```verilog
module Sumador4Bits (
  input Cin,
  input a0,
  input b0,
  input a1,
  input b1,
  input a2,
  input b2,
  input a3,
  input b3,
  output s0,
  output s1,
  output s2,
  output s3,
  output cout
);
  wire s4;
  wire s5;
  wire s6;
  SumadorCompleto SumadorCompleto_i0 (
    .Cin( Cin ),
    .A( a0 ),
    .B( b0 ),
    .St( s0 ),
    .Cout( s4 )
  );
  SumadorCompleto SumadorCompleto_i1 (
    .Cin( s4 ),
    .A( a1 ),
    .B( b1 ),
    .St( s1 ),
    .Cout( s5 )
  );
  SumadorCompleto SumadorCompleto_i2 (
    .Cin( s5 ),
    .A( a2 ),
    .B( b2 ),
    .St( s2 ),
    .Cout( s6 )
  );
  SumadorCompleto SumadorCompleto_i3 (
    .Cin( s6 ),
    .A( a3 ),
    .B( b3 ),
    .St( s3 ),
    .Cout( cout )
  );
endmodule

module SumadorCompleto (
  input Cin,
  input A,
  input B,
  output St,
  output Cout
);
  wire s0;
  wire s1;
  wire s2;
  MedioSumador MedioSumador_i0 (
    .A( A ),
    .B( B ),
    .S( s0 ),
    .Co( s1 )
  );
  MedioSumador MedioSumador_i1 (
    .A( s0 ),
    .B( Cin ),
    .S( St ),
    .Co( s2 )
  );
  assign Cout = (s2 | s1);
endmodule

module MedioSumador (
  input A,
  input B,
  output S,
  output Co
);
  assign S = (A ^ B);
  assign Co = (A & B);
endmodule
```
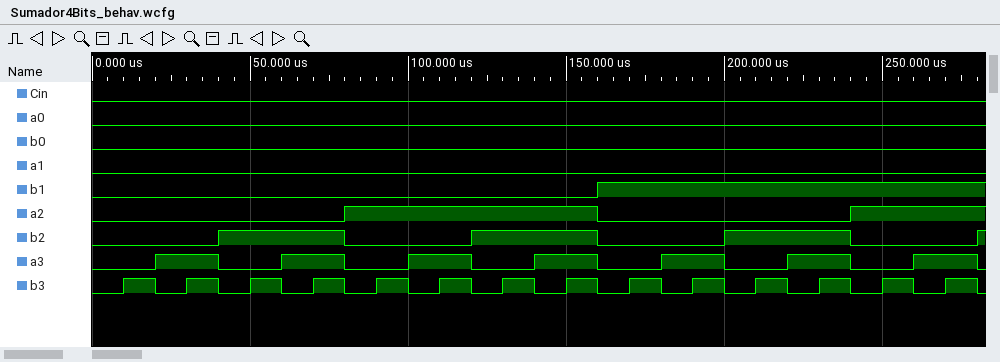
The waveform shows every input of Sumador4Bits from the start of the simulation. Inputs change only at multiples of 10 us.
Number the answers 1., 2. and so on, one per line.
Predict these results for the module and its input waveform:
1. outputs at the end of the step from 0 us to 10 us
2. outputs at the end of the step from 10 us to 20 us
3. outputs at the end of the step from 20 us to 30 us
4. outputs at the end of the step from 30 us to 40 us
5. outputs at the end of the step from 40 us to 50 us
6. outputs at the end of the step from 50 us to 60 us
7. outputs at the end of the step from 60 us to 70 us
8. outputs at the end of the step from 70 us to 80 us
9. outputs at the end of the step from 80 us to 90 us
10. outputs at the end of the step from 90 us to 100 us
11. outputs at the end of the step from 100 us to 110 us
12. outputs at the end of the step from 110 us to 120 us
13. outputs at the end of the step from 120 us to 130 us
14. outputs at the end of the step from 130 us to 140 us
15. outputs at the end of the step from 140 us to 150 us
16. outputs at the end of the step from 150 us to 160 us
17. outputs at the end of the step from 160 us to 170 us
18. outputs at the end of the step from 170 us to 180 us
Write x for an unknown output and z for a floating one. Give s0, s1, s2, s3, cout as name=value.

1. s0=0, s1=0, s2=0, s3=0, cout=0
2. s0=0, s1=0, s2=0, s3=1, cout=0
3. s0=0, s1=0, s2=0, s3=1, cout=0
4. s0=0, s1=0, s2=0, s3=0, cout=1
5. s0=0, s1=0, s2=1, s3=0, cout=0
6. s0=0, s1=0, s2=1, s3=1, cout=0
7. s0=0, s1=0, s2=1, s3=1, cout=0
8. s0=0, s1=0, s2=1, s3=0, cout=1
9. s0=0, s1=0, s2=1, s3=0, cout=0
10. s0=0, s1=0, s2=1, s3=1, cout=0
11. s0=0, s1=0, s2=1, s3=1, cout=0
12. s0=0, s1=0, s2=1, s3=0, cout=1
13. s0=0, s1=0, s2=0, s3=1, cout=0
14. s0=0, s1=0, s2=0, s3=0, cout=1
15. s0=0, s1=0, s2=0, s3=0, cout=1
16. s0=0, s1=0, s2=0, s3=1, cout=1
17. s0=0, s1=1, s2=0, s3=0, cout=0
18. s0=0, s1=1, s2=0, s3=1, cout=0
